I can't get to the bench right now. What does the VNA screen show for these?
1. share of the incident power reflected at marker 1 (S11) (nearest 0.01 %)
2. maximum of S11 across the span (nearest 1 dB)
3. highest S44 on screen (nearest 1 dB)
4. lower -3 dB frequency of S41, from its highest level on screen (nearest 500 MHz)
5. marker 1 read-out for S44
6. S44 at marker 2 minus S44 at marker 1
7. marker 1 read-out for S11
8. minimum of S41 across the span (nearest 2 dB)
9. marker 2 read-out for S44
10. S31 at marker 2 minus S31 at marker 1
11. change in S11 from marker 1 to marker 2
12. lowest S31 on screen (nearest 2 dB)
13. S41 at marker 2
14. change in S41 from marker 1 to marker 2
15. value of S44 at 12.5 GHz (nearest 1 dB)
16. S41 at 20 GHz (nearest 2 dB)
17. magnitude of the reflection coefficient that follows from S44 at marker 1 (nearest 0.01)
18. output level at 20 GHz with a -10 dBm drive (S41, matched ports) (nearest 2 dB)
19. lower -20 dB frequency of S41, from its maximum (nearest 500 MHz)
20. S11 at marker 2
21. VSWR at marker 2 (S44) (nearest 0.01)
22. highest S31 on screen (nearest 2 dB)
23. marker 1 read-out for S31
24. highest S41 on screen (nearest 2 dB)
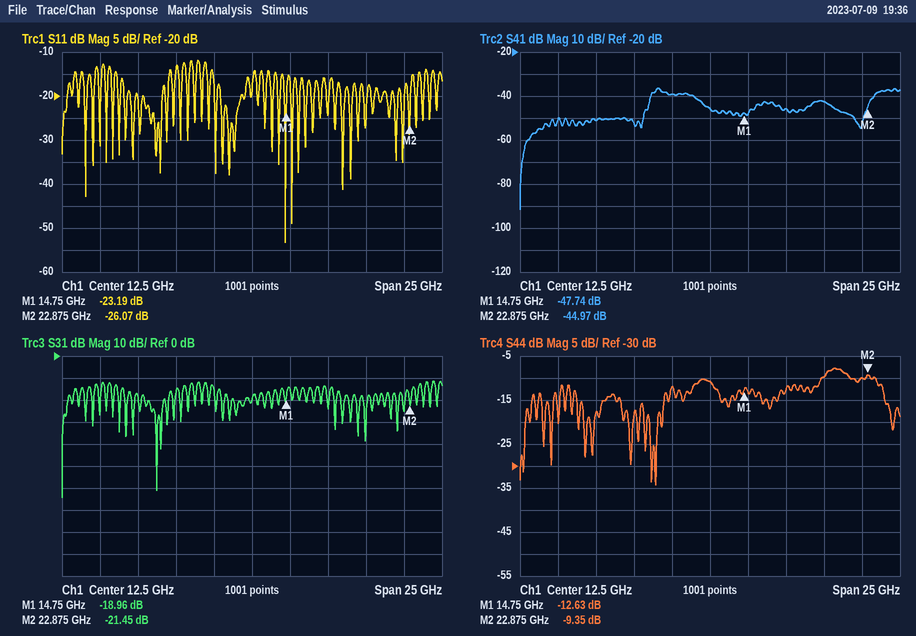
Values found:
0.48 %
-12 dB
-8 dB
8.5 GHz
-12.63 dB
3.28 dB
-23.19 dB
-92 dB
-9.35 dB
-2.49 dB
-2.88 dB
-64 dB
-44.97 dB
2.77 dB
-11 dB
-42 dB
0.23
-52 dBm
1.0 GHz
-26.07 dB
2.03
-12 dB
-18.96 dB
-36 dB
